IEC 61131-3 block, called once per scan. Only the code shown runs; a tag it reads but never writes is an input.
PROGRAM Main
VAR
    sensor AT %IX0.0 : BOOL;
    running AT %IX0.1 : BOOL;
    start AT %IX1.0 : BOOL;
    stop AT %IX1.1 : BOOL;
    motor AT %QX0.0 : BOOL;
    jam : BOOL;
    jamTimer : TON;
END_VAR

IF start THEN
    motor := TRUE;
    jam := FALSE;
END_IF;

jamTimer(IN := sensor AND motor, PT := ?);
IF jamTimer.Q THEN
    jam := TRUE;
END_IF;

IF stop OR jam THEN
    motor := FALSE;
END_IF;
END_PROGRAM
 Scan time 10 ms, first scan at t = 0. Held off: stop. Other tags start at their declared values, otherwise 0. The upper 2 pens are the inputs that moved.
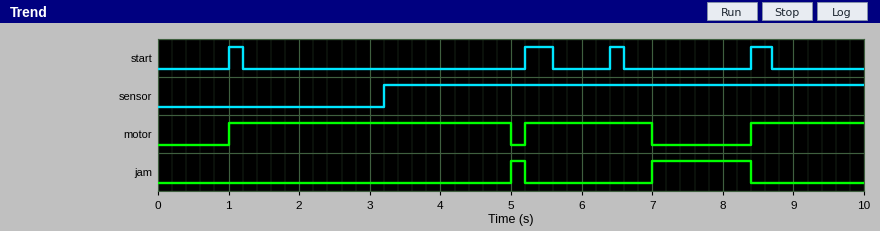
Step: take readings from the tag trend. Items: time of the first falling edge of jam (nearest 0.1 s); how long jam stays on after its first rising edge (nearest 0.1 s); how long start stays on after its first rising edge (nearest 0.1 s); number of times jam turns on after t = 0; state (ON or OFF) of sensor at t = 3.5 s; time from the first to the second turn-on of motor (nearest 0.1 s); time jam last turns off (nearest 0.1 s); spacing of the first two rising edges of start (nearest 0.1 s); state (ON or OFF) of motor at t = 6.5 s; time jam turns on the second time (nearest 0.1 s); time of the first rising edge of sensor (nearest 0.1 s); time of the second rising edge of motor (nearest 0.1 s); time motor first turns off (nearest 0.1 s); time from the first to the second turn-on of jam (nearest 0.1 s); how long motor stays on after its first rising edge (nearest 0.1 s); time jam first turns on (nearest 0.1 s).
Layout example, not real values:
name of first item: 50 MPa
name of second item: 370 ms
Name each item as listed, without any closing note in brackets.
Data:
time of the first falling edge of jam: 5.2 s
how long jam stays on after its first rising edge: 0.2 s
how long start stays on after its first rising edge: 0.2 s
number of times jam turns on after t = 0: 2
state (ON or OFF) of sensor at t = 3.5 s: ON
time from the first to the second turn-on of motor: 4.2 s
time jam last turns off: 8.4 s
spacing of the first two rising edges of start: 4.2 s
state (ON or OFF) of motor at t = 6.5 s: ON
time jam turns on the second time: 7.0 s
time of the first rising edge of sensor: 3.2 s
time of the second rising edge of motor: 5.2 s
time motor first turns off: 5.0 s
time from the first to the second turn-on of jam: 2.0 s
how long motor stays on after its first rising edge: 4.0 s
time jam first turns on: 5.0 s
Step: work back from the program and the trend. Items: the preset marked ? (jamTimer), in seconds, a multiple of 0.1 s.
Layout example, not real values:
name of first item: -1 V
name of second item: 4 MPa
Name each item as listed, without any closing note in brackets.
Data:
the preset marked ? (jamTimer), in seconds, a multiple of 0.1 s: 1.8 s
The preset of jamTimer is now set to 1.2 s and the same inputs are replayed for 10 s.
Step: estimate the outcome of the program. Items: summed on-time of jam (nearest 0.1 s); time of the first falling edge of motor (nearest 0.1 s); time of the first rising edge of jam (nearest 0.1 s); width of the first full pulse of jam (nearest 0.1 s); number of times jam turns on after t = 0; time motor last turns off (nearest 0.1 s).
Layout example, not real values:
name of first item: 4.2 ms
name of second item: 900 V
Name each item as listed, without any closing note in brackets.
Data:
summed on-time of jam: 3.2 s
time of the first falling edge of motor: 4.4 s
time of the first rising edge of jam: 4.4 s
width of the first full pulse of jam: 0.8 s
number of times jam turns on after t = 0: 3
time motor last turns off: 9.6 s
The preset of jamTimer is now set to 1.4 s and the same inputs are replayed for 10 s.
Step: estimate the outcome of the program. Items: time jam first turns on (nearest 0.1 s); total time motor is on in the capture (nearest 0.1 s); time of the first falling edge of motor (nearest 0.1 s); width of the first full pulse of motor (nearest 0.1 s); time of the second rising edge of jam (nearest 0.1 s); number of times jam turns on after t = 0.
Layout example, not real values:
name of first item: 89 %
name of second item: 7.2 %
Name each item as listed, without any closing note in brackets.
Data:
time jam first turns on: 4.6 s
total time motor is on in the capture: 6.4 s
time of the first falling edge of motor: 4.6 s
width of the first full pulse of motor: 3.6 s
time of the second rising edge of jam: 6.6 s
number of times jam turns on after t = 0: 3
